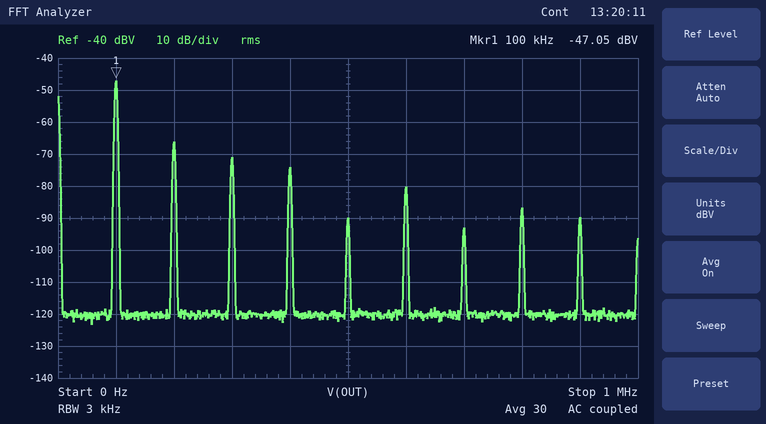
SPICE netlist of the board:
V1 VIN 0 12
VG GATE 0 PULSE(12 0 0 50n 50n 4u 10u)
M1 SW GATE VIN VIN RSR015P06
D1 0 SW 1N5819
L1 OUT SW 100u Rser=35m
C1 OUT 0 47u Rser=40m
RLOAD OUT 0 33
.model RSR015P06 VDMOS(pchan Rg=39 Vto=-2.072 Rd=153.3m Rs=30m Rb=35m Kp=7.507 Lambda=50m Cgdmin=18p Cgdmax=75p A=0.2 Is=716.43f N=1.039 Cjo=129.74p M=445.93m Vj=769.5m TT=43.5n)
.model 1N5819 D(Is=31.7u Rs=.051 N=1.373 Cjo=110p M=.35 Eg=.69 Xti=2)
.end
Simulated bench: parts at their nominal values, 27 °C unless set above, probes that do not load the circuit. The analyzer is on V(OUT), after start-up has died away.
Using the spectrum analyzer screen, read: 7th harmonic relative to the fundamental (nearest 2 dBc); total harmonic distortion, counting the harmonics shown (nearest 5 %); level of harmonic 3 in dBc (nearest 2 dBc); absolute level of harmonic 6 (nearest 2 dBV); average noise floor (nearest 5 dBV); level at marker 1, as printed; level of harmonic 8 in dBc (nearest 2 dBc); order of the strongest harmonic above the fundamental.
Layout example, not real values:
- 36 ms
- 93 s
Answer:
- -46 dBc
- 15 %
- -24 dBc
- -80 dBV
- -120 dBV
- -47.05 dBV
- -40 dBc
- 2
